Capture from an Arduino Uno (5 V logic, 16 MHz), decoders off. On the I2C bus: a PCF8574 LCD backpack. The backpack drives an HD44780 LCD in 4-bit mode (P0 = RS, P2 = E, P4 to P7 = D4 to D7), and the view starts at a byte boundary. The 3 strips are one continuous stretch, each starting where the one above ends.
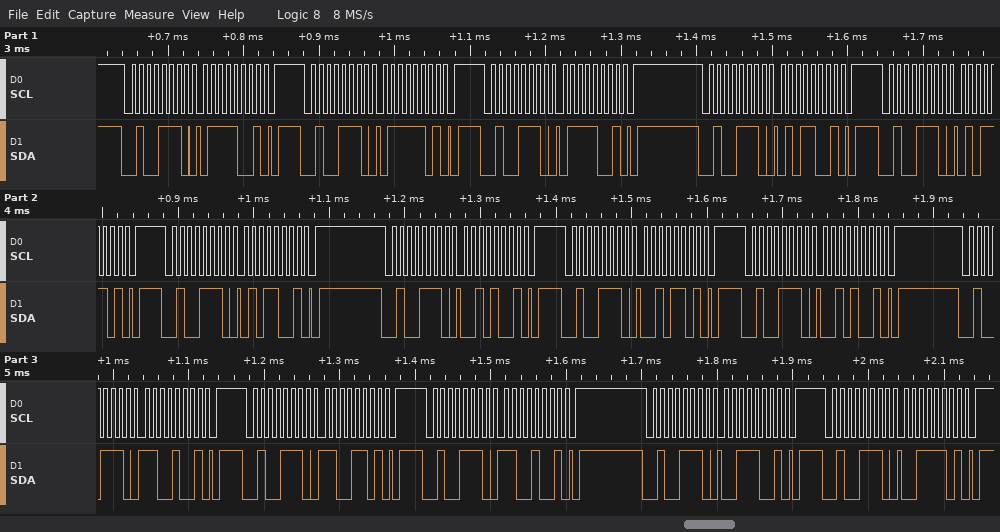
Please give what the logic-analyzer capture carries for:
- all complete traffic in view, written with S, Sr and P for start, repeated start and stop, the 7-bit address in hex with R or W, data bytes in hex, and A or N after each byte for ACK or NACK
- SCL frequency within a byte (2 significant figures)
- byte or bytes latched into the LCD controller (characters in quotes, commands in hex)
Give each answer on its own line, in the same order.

S 27W A 79 A P S 27W A 7D A P S 27W A 79 A P S 27W A 59 A P S 27W A 5D A P S 27W A 59 A P S 27W A 29 A P S 27W A 2D A P S 27W A 29 A P S 27W A C9 A P S 27W A CD A P S 27W A C9 A P S 27W A 39 A P S 27W A 3D A P
100 kHz
'u' ','
